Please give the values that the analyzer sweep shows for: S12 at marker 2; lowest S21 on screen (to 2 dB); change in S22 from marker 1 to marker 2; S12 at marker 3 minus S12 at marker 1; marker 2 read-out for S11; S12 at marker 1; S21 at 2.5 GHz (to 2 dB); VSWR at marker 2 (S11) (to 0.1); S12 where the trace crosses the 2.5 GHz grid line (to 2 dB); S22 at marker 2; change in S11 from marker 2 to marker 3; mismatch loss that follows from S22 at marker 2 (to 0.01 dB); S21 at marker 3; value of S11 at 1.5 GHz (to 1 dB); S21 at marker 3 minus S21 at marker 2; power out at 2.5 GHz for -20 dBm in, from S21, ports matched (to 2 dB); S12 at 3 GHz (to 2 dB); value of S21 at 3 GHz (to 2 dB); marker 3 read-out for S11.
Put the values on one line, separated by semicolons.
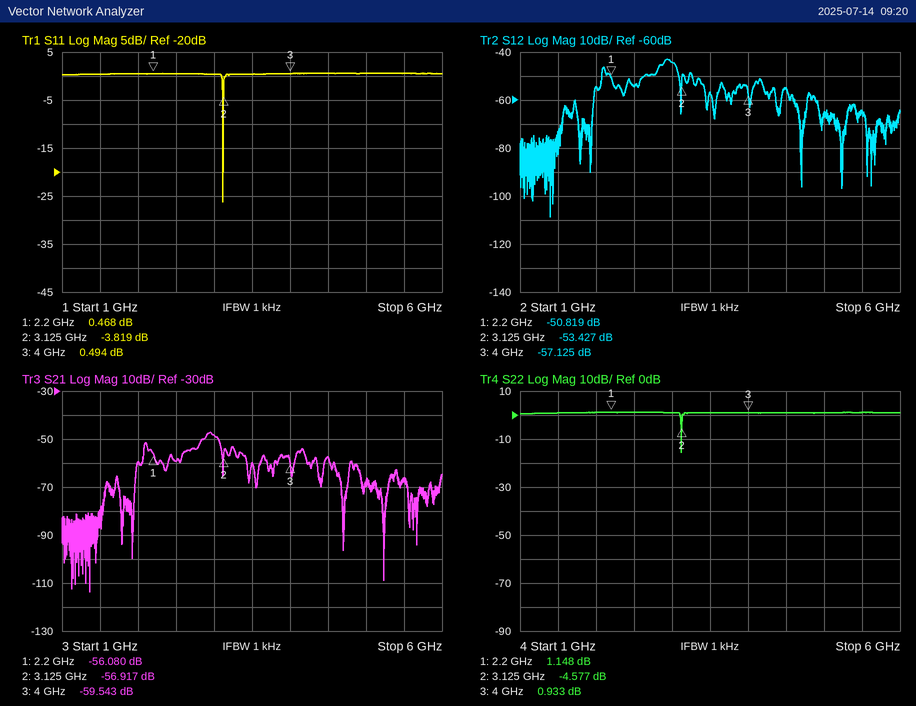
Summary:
-53.427 dB; -114 dB; -5.725 dB; -6.306 dB; -3.819 dB; -50.819 dB; -60 dB; 4.6; -54 dB; -4.577 dB; 4.313 dB; 1.86 dB; -59.543 dB; 0 dB; -2.626 dB; -80 dBm; -44 dB; -48 dB; 0.494 dB
